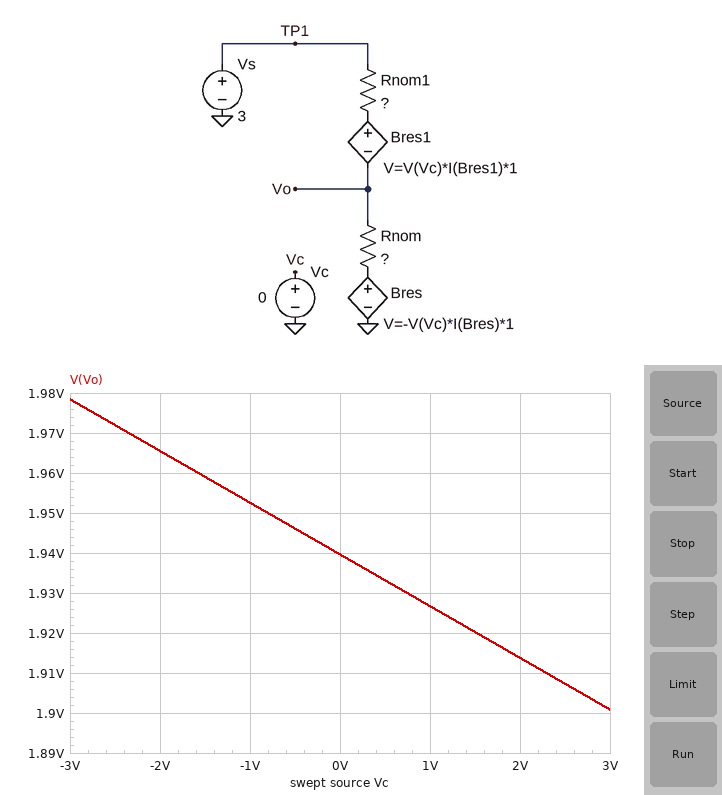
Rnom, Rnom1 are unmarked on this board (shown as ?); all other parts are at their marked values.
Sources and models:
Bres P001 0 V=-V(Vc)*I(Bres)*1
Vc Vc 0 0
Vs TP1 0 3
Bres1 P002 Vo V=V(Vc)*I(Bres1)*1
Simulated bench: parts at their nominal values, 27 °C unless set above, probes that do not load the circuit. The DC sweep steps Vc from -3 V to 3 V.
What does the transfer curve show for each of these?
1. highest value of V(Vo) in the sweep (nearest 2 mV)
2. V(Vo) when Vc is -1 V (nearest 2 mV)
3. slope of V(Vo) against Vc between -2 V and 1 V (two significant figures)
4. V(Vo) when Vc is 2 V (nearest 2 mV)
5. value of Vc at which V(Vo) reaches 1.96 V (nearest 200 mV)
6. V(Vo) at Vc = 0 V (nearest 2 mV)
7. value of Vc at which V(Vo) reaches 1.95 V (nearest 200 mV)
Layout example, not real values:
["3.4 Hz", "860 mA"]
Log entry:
["1.978 V", "1.952 V", "-0.013 V/V", "1.914 V", "-1.6 V", "1.940 V", "-800 mV"]
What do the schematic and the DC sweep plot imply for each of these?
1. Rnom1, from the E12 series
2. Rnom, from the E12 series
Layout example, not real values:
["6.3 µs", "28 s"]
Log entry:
["82 Ω", "150 Ω"]
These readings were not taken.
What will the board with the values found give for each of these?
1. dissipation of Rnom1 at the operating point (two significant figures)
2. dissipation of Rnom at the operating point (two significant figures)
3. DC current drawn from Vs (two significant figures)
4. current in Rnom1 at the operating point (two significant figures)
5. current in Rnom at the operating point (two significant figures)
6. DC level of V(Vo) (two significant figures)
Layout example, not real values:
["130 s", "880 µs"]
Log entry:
["14 mW", "25 mW", "13 mA", "13 mA", "13 mA", "1.9 V"]
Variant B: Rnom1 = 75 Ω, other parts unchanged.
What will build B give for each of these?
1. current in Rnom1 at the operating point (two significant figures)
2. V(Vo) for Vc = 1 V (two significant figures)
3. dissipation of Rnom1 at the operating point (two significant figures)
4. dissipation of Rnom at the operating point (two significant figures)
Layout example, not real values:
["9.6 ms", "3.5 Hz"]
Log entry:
["13 mA", "2.0 V", "13 mW", "27 mW"]
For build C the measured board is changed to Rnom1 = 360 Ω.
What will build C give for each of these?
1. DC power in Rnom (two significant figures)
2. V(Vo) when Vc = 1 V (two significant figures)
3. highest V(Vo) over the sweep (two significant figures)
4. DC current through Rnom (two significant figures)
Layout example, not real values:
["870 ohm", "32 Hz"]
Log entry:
["5.2 mW", "880 mV", "900 mV", "5.9 mA"]
